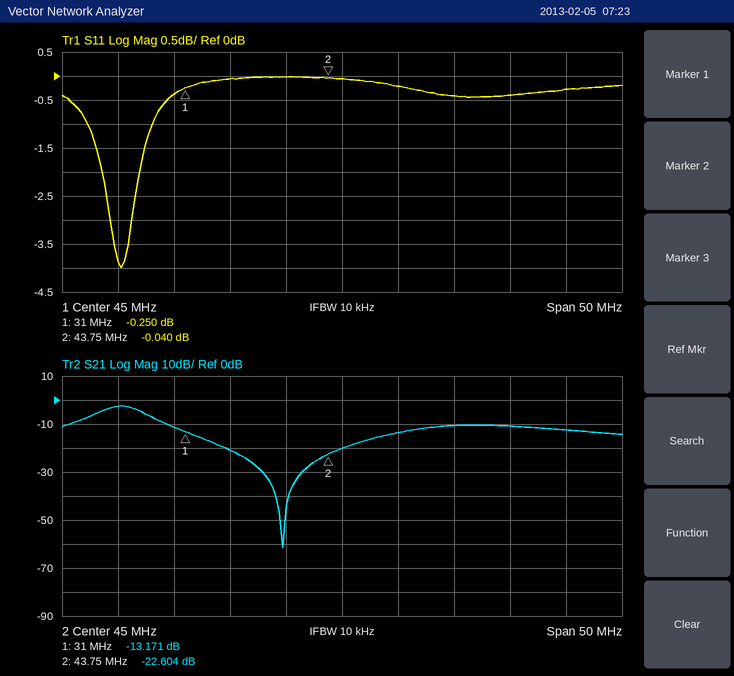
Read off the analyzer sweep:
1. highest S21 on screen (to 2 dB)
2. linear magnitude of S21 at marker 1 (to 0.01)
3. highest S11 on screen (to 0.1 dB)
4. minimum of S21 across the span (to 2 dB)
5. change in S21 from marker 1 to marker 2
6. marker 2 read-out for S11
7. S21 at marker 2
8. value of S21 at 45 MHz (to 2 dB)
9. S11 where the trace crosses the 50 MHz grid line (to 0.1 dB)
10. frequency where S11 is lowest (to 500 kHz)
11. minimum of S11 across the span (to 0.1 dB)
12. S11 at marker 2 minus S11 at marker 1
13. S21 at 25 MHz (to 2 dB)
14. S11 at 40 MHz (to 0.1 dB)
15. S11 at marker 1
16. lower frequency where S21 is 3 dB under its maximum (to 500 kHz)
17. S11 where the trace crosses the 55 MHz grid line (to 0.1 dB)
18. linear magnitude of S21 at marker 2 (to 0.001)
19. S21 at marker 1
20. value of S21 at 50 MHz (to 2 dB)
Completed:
-2 dB
0.22
0.0 dB
-62 dB
-9.433 dB
-0.040 dB
-22.604 dB
-20 dB
-0.2 dB
25.5 MHz
-4.0 dB
0.210 dB
-2 dB
0.0 dB
-0.250 dB
23.0 MHz
-0.4 dB
0.074
-13.171 dB
-14 dB
